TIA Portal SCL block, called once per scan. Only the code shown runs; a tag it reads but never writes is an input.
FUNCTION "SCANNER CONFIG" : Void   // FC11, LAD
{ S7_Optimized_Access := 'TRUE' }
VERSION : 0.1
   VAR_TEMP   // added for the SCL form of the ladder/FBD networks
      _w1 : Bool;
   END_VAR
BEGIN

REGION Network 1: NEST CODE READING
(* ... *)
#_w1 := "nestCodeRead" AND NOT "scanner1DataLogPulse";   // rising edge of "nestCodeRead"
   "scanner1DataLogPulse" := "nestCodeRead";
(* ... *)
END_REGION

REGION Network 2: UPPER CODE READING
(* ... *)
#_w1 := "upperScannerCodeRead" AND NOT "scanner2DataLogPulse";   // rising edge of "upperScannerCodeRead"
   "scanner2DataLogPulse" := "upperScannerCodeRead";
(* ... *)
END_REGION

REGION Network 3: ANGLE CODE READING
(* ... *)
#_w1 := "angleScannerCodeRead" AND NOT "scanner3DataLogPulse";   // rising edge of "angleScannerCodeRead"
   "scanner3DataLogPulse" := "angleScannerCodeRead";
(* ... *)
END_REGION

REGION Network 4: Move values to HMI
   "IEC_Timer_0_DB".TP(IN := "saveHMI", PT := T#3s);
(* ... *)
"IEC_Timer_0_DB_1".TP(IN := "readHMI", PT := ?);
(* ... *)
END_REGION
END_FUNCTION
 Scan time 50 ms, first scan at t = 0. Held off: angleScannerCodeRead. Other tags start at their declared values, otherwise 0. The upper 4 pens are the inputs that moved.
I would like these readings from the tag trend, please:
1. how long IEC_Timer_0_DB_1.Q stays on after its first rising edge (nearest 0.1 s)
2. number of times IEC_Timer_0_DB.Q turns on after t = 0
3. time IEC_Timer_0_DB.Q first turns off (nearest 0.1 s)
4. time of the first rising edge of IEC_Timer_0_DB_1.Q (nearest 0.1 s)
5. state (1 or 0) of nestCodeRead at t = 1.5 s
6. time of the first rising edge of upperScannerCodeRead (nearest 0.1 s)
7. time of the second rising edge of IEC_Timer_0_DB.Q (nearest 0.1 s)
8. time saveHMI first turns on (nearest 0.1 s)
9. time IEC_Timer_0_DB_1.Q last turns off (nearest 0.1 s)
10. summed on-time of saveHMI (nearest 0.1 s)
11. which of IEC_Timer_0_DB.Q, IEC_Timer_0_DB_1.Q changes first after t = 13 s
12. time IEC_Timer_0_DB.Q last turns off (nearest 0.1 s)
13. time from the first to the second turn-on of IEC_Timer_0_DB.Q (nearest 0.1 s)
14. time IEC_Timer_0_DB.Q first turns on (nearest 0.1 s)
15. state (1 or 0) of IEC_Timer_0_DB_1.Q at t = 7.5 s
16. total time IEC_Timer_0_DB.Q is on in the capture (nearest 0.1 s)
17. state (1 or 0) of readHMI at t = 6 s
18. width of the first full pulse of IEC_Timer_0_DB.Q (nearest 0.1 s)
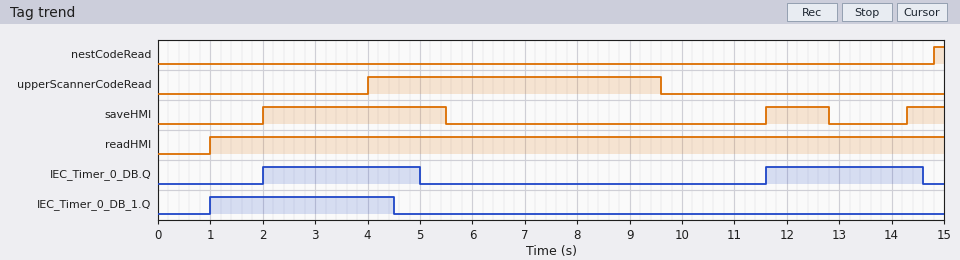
3.5 s
2
5.0 s
1.0 s
0
4.0 s
11.6 s
2.0 s
4.5 s
5.4 s
IEC_Timer_0_DB.Q
14.6 s
9.6 s
2.0 s
0
6.0 s
1
3.0 s
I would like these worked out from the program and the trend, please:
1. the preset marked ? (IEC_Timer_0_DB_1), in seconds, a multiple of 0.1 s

3.5 s
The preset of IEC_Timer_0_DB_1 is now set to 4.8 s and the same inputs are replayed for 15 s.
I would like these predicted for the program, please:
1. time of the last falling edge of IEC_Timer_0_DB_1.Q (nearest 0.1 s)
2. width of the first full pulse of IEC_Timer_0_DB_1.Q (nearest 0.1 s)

5.8 s
4.8 s
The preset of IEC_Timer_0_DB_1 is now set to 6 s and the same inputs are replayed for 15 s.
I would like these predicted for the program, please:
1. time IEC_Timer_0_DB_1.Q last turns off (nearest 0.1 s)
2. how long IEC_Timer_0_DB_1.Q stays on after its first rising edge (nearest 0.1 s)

7.0 s
6.0 s
